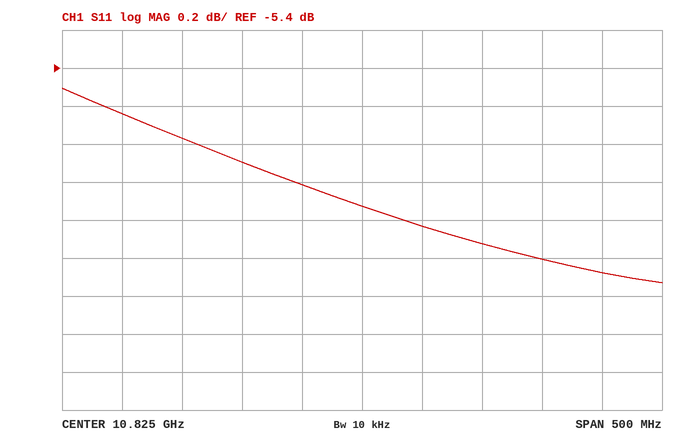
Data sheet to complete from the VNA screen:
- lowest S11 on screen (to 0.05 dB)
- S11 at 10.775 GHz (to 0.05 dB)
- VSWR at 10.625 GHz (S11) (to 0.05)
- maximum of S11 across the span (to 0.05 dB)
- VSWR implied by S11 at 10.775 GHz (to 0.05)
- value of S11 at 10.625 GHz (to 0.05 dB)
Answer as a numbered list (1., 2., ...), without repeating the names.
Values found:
1. -6.55 dB
2. -6.00 dB
3. 3.20
4. -5.50 dB
5. 3.00
6. -5.65 dB
